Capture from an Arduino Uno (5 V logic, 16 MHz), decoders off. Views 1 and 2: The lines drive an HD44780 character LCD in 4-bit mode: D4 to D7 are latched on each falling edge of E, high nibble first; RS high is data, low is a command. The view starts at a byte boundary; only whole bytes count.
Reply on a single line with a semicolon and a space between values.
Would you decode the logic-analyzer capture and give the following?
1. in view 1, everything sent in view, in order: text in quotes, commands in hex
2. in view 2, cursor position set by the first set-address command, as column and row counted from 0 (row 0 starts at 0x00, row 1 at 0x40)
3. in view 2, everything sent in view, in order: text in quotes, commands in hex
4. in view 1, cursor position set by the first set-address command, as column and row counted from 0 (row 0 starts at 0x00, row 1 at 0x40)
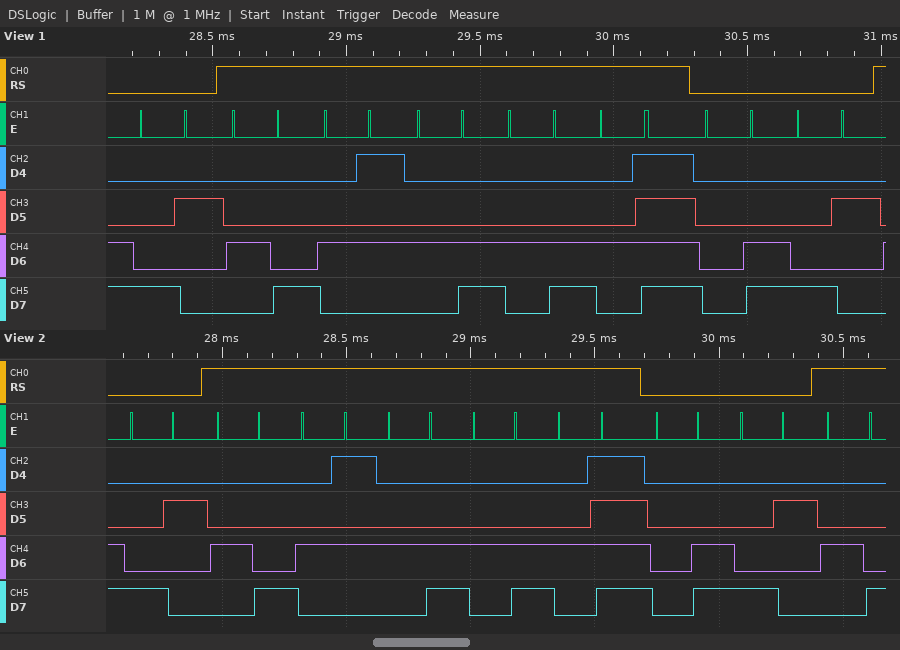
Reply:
0x82 "HELLO" 0x0C 0x82; column 2, row 0; 0x82 "HELLO" 0x0C 0x82 "H"; column 2, row 0
